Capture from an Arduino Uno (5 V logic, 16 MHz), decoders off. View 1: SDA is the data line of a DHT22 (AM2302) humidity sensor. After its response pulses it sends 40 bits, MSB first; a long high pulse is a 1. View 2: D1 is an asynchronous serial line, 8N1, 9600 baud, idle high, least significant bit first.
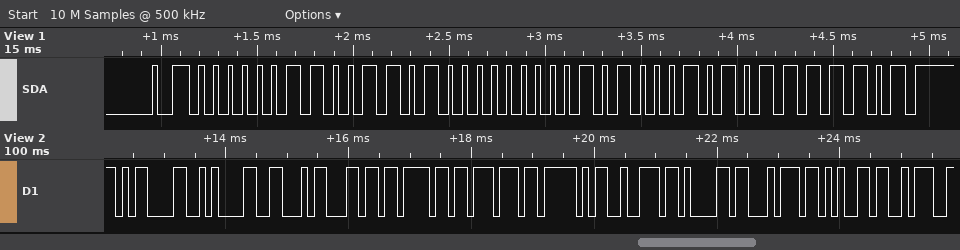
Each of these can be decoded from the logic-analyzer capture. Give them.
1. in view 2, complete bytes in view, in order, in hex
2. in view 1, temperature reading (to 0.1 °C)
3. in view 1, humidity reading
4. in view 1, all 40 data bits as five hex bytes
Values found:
0x0D 0x0A 0x46 0x6C 0x6F 0x77 0x5F 0x72 0x61 0x74 0x65 0x3A
32.5 °C
82.0 %
03 34 01 45 7D
